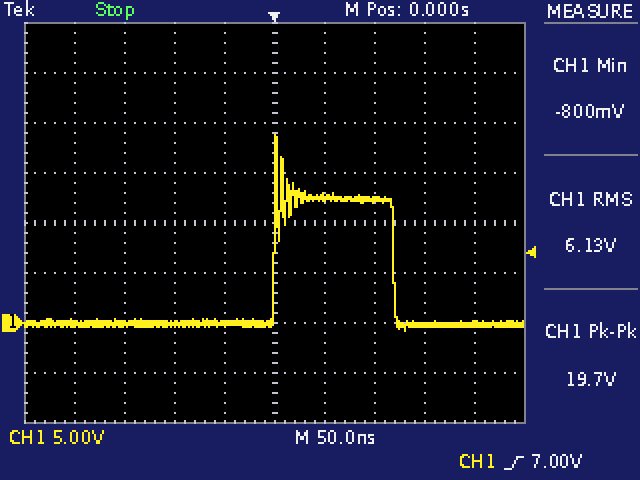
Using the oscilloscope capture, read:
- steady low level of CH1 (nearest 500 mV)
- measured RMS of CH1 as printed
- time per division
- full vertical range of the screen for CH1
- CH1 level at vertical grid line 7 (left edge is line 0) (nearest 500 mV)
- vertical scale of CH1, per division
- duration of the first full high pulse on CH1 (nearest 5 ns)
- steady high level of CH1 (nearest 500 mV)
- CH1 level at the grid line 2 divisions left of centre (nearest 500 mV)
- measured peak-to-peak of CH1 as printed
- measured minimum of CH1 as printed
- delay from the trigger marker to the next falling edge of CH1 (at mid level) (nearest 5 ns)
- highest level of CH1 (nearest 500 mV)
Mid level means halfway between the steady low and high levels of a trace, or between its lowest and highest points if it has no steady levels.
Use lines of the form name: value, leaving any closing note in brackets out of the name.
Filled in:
steady low level of CH1: 0.0 V
measured RMS of CH1 as printed: 6.13 V
time per division: 50 ns
full vertical range of the screen for CH1: 40 V
CH1 level at vertical grid line 7 (left edge is line 0): 12.5 V
vertical scale of CH1, per division: 5 V
duration of the first full high pulse on CH1: 120 ns
steady high level of CH1: 12.5 V
CH1 level at the grid line 2 divisions left of centre: 0.0 V
measured peak-to-peak of CH1 as printed: 19.7 V
measured minimum of CH1 as printed: -800 mV
delay from the trigger marker to the next falling edge of CH1 (at mid level): 120 ns
highest level of CH1: 19.0 V
